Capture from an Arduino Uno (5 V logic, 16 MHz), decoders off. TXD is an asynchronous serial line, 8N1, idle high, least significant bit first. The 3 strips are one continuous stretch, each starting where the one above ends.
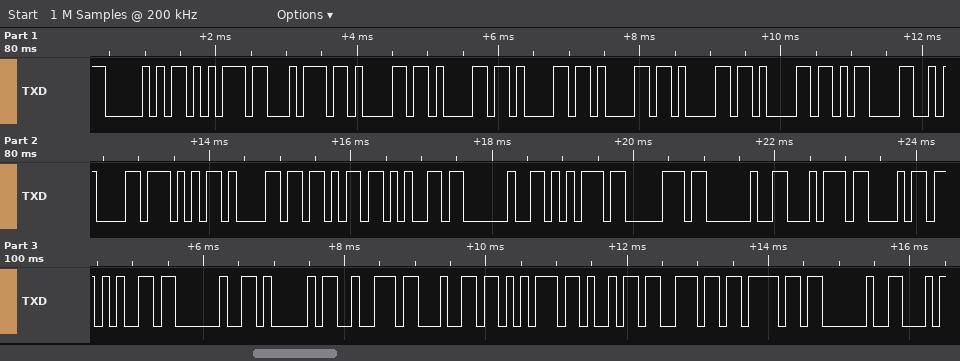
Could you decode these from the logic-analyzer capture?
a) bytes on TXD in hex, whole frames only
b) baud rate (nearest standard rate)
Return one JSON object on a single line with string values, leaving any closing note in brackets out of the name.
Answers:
{"bytes on TXD in hex, whole frames only": "0x50 0x75 0x74 0x61 0x61 0x61 0x61 0x61 0x61 0x0D 0x0A 0x57 0x61 0x6B 0x65 0x20 0x75 0x70 0x20 0x74 0x68 0x65 0x20 0x41 0x72 0x64 0x75 0x69 0x6E 0x6F 0x20", "baud rate": "9600 baud"}
